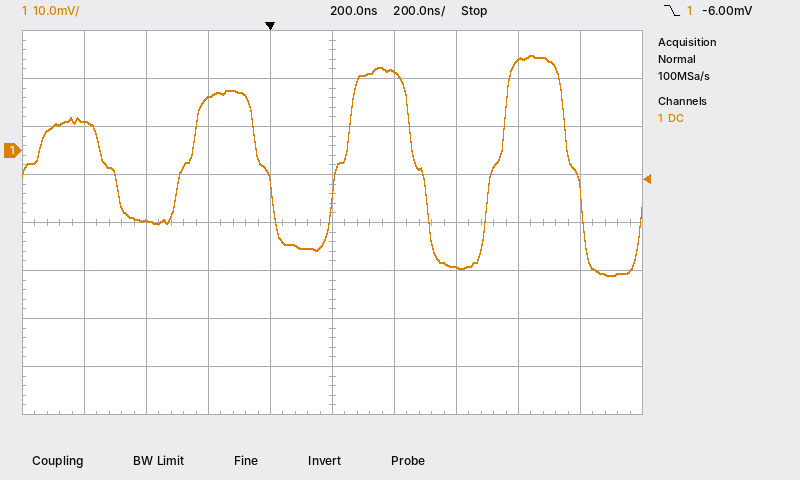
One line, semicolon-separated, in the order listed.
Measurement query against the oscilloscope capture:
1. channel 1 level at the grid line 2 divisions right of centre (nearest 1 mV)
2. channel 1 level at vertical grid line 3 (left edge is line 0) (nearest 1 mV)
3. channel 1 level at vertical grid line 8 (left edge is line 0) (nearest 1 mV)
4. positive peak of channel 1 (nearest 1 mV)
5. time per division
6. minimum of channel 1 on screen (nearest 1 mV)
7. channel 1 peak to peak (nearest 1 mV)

-24 mV; 11 mV; 19 mV; 20 mV; 200 ns; -26 mV; 46 mV
